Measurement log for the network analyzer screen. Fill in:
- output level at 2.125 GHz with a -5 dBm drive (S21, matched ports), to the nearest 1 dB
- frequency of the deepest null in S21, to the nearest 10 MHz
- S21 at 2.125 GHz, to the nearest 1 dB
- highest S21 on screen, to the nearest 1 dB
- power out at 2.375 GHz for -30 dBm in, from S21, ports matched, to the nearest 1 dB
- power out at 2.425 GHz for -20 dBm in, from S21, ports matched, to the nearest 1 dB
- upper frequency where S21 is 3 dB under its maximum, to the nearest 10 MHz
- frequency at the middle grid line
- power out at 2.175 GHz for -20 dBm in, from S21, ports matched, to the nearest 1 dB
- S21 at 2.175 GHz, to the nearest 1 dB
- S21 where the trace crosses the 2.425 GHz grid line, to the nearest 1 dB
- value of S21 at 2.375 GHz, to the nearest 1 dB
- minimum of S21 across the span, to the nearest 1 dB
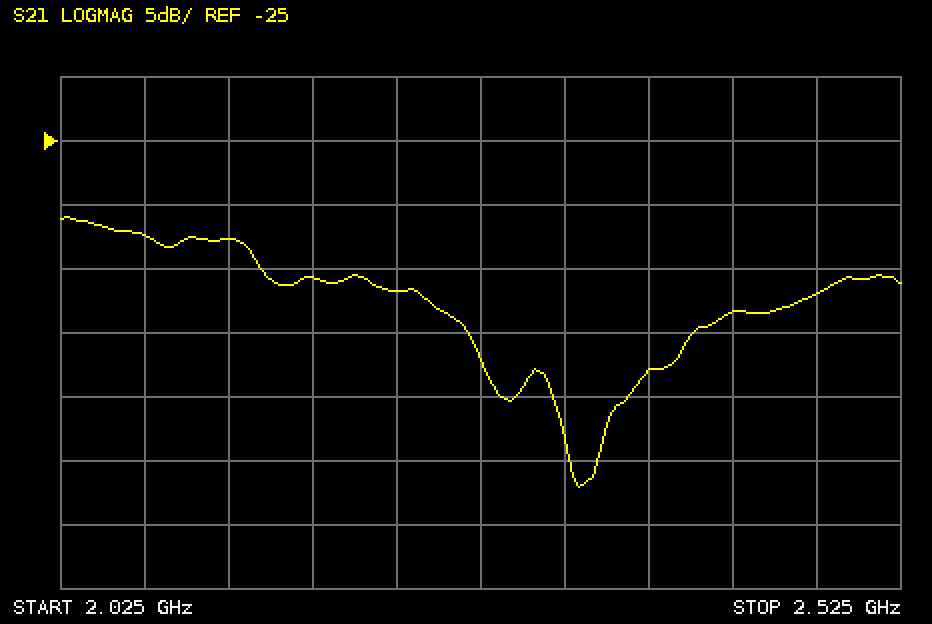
-38 dBm
2.33 GHz
-33 dB
-31 dB
-73 dBm
-58 dBm
2.14 GHz
2.275 GHz
-56 dBm
-36 dB
-38 dB
-43 dB
-52 dB
